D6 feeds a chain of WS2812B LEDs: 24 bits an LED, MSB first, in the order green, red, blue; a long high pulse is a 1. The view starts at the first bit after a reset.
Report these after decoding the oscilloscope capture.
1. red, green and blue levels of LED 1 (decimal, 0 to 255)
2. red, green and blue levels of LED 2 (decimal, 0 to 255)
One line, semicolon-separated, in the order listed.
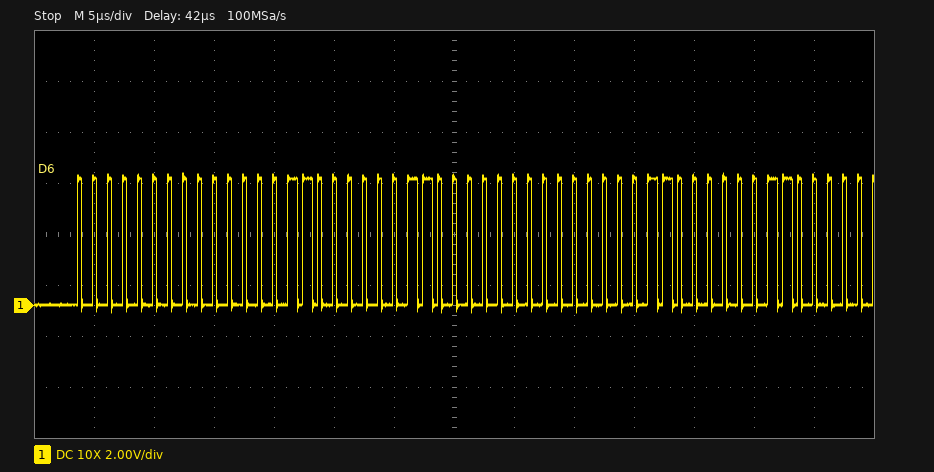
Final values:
3, 0, 3; 3, 0, 3
